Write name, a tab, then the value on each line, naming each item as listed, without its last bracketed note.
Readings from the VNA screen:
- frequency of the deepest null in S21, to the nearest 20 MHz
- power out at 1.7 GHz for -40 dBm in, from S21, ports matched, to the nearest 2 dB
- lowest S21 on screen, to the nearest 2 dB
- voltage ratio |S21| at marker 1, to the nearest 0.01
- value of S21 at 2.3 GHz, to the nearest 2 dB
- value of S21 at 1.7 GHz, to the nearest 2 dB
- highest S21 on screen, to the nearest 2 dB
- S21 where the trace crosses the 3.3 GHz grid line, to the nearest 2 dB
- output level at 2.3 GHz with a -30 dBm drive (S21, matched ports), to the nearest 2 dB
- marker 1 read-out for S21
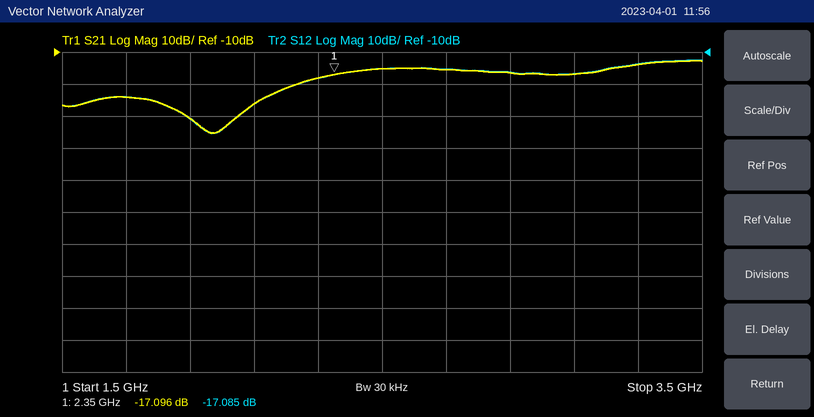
frequency of the deepest null in S21, to the nearest 20 MHz	1.96 GHz
power out at 1.7 GHz for -40 dBm in, from S21, ports matched, to the nearest 2 dB	-64 dBm
lowest S21 on screen, to the nearest 2 dB	-36 dB
voltage ratio |S21| at marker 1, to the nearest 0.01	0.14
value of S21 at 2.3 GHz, to the nearest 2 dB	-18 dB
value of S21 at 1.7 GHz, to the nearest 2 dB	-24 dB
highest S21 on screen, to the nearest 2 dB	-12 dB
S21 where the trace crosses the 3.3 GHz grid line, to the nearest 2 dB	-14 dB
output level at 2.3 GHz with a -30 dBm drive (S21, matched ports), to the nearest 2 dB	-48 dBm
marker 1 read-out for S21	-17.096 dB
